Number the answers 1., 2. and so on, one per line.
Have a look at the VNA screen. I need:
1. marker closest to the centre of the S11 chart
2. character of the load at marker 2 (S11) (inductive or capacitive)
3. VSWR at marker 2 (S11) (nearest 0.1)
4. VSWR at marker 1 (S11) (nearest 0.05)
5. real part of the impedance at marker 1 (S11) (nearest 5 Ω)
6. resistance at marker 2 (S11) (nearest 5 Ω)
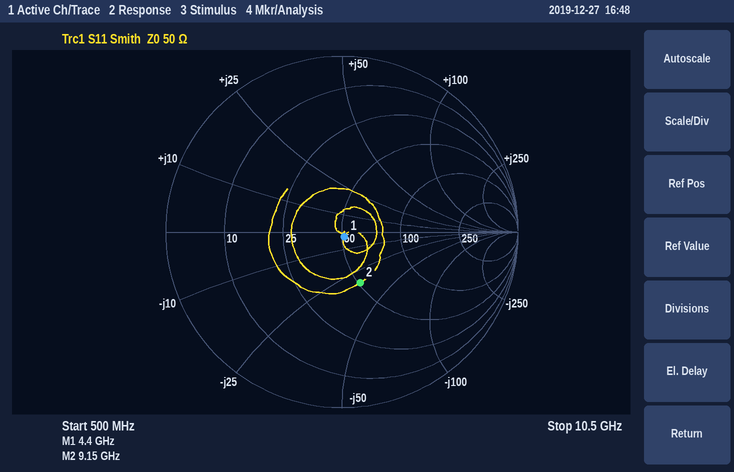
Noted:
1. marker 1
2. capacitive
3. 1.9
4. 1.05
5. 50 Ω
6. 50 Ω
